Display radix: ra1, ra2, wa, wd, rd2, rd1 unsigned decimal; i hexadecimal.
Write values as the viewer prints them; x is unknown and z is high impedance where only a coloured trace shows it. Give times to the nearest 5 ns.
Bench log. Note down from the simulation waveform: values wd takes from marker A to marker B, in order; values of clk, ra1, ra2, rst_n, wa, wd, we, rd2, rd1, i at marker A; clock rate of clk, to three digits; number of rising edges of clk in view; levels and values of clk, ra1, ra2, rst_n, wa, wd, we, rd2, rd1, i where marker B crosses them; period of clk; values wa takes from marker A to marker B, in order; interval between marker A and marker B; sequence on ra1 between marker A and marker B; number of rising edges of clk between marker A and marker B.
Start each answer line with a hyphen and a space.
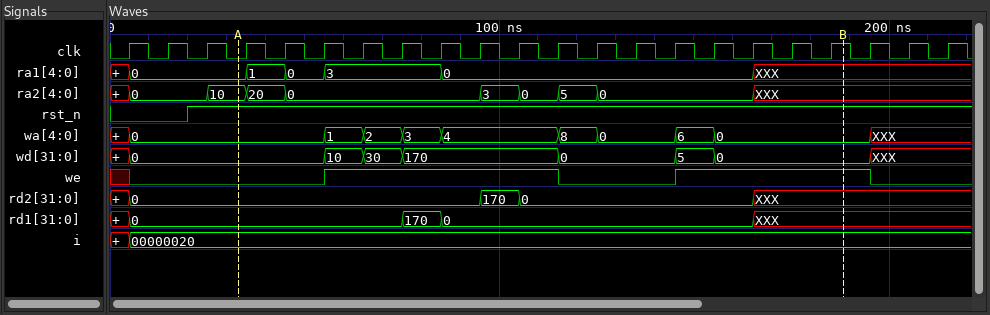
- 0, 10, 30, 170, 0, 5, 0
- clk=0, ra1=0, ra2=10, rst_n=1, wa=0, wd=0, we=0, rd2=0, rd1=0, i=00000020
- 100 MHz
- 22
- clk=1, ra1=XXX, ra2=XXX, rst_n=1, wa=0, wd=0, we=1, rd2=XXX, rd1=XXX, i=00000020
- 10 ns
- 0, 1, 2, 3, 4, 8, 0, 6, 0
- 155 ns
- 0, 1, 0, 3, 0, XXX
- 16
